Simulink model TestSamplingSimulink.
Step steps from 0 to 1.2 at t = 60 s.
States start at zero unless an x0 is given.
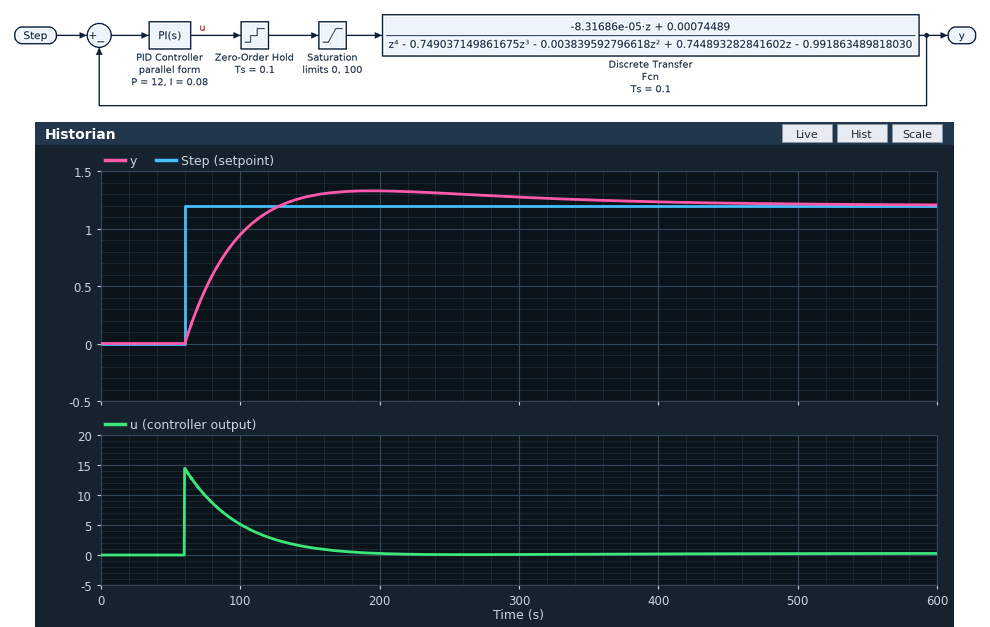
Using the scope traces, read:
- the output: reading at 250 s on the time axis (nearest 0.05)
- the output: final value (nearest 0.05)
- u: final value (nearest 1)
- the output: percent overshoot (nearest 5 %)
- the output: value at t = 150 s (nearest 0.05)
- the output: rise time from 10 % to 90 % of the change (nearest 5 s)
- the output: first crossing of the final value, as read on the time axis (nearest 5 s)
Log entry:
1.30
1.20
0
10 %
1.30
50 s
130 s
